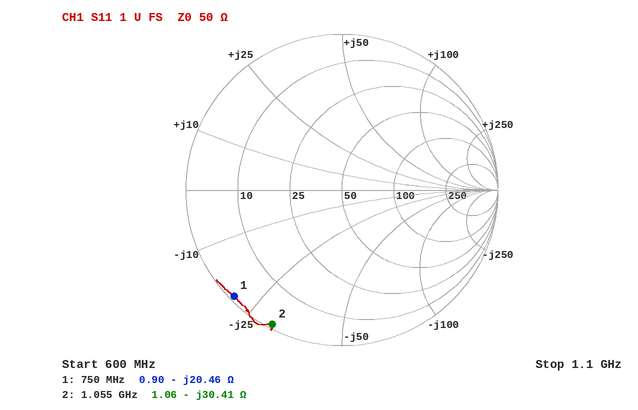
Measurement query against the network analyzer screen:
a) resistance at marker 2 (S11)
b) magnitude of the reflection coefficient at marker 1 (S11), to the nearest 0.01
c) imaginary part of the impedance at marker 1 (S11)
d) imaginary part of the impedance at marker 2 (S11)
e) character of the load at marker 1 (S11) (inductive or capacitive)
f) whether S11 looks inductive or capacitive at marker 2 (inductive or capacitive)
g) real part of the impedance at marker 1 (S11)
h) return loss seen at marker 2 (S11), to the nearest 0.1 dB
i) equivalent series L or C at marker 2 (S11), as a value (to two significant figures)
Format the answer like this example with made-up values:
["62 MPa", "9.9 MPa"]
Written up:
["1.06 Ω", "0.97", "-20.46 Ω", "-30.41 Ω", "capacitive", "capacitive", "0.90 Ω", "0.3 dB", "5.0 pF"]
